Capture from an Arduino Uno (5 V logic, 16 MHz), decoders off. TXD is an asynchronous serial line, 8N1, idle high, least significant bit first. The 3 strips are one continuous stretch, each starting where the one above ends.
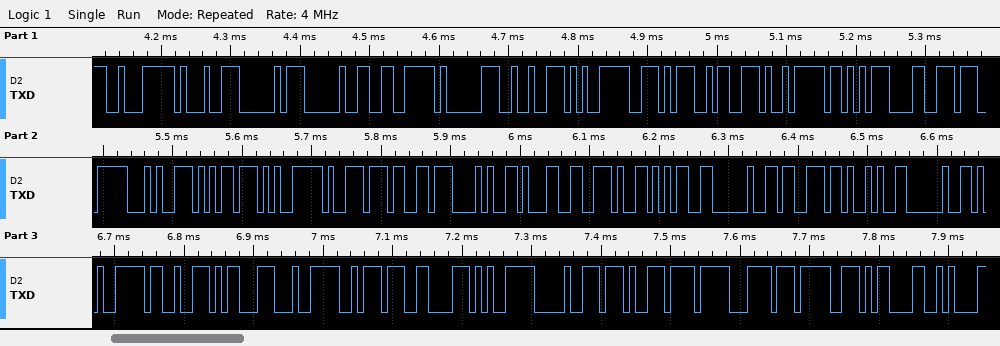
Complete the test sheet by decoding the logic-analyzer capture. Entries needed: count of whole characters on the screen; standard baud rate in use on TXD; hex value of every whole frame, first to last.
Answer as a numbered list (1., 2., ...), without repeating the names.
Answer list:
1. 41
2. 115200 baud
3. 0xE2 0x91 0xA0 0x20 0xE6 0x81 0x92 0xE5 0xAE 0x9A 0xE9 0xAB 0x98 0xE7 0x94 0xB5 0xE5 0xB9 0xB3 0x28 0x31 0x2E 0x35 0x20 0x73 0x29 0x20 0xE5 0x93 0x8D 0xE4 0xBA 0x86 0xE5 0x90 0x97 0xEF 0xBC 0x9F 0x0D 0x0A
